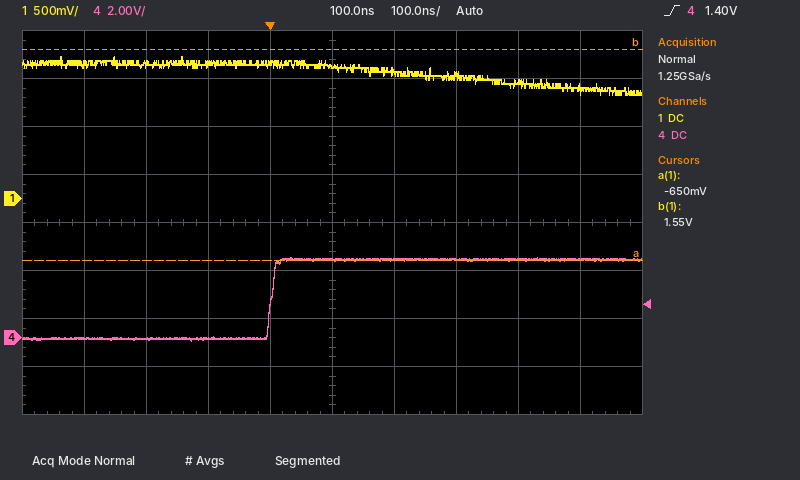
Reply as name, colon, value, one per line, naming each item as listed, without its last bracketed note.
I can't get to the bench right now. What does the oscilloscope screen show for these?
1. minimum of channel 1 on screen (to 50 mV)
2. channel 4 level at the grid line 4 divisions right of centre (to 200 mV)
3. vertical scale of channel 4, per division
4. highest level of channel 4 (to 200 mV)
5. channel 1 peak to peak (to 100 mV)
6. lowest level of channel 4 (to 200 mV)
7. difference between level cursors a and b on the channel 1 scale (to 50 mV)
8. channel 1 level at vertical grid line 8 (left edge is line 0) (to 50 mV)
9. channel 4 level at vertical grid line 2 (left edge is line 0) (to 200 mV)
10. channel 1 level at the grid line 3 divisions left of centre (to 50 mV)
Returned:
minimum of channel 1 on screen: 1.10 V
channel 4 level at the grid line 4 divisions right of centre: 3.2 V
vertical scale of channel 4, per division: 2 V
highest level of channel 4: 3.4 V
channel 1 peak to peak: 400 mV
lowest level of channel 4: -200 mV
difference between level cursors a and b on the channel 1 scale: 2.20 V
channel 1 level at vertical grid line 8 (left edge is line 0): 1.20 V
channel 4 level at vertical grid line 2 (left edge is line 0): 0.0 V
channel 1 level at the grid line 3 divisions left of centre: 1.40 V
